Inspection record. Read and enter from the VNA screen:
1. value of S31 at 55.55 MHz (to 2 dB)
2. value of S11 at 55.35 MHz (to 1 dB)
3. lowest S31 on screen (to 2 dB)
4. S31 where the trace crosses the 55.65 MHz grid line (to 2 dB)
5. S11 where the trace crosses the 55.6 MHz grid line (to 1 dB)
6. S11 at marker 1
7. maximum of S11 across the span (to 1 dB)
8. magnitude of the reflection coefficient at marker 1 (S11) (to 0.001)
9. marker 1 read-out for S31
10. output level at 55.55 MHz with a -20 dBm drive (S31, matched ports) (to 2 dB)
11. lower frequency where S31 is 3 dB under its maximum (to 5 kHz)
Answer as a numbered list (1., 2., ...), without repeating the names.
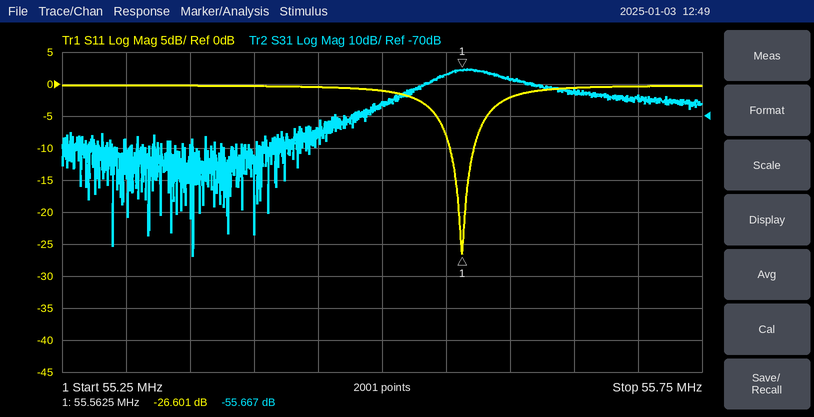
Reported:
1. -58 dB
2. 0 dB
3. -114 dB
4. -62 dB
5. -2 dB
6. -26.601 dB
7. 0 dB
8. 0.047
9. -55.667 dB
10. -78 dBm
11. 55.545 MHz
